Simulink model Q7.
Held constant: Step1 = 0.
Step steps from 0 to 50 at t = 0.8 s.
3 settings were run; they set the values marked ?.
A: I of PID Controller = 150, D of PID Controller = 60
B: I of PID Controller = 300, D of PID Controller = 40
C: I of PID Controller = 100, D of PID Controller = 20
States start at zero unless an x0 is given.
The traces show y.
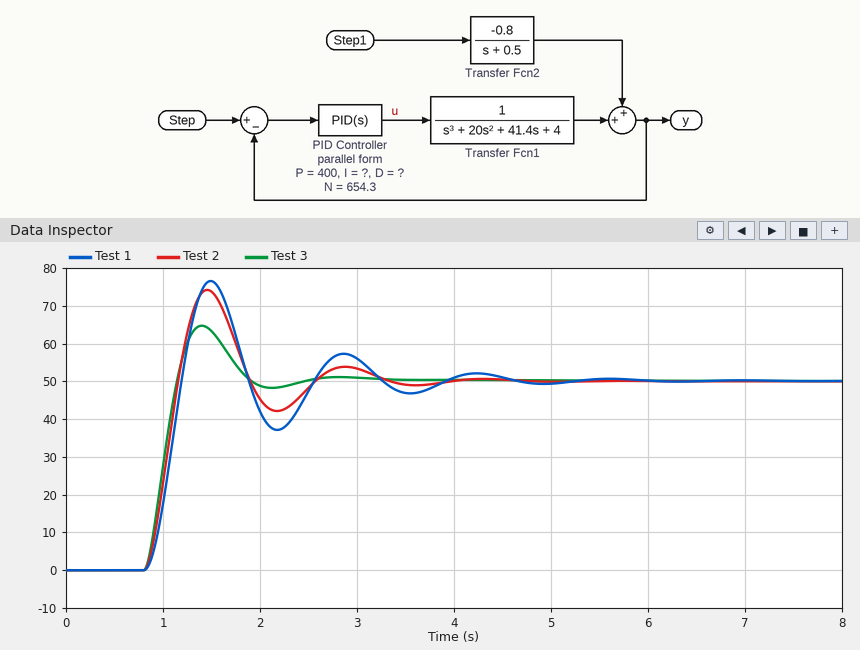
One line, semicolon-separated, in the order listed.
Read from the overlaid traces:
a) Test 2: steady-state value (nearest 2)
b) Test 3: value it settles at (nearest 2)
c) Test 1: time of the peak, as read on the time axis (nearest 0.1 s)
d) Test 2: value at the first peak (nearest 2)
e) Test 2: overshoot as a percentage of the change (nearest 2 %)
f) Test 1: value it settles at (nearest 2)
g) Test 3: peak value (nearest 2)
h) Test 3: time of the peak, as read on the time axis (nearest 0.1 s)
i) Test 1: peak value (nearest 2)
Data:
50; 50; 1.5 s; 74; 48 %; 50; 64; 1.4 s; 76
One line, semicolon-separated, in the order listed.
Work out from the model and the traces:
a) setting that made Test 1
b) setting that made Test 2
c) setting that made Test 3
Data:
C; B; A
